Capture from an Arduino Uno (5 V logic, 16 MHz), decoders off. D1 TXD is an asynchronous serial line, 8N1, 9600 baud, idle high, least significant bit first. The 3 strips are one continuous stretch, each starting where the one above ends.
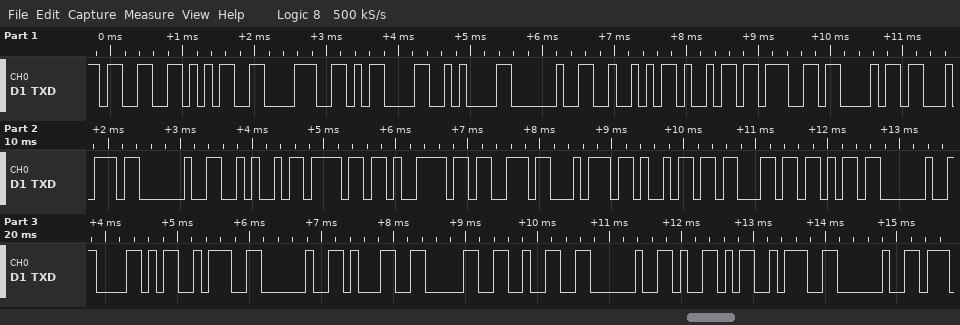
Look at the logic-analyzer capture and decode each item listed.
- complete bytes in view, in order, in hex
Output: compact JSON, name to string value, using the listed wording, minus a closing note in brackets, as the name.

{"complete bytes in view, in order, in hex": "0x33 0x35 0x38 0x0D 0x0A 0x20 0x52 0x69 0x67 0x68 0x74 0x20 0x4A 0x6F 0x79 0x73 0x74 0x69 0x63 0x6B 0x20 0x58 0x3A 0x20 0x31 0x30 0x32 0x20 0x59 0x3A 0x20"}
